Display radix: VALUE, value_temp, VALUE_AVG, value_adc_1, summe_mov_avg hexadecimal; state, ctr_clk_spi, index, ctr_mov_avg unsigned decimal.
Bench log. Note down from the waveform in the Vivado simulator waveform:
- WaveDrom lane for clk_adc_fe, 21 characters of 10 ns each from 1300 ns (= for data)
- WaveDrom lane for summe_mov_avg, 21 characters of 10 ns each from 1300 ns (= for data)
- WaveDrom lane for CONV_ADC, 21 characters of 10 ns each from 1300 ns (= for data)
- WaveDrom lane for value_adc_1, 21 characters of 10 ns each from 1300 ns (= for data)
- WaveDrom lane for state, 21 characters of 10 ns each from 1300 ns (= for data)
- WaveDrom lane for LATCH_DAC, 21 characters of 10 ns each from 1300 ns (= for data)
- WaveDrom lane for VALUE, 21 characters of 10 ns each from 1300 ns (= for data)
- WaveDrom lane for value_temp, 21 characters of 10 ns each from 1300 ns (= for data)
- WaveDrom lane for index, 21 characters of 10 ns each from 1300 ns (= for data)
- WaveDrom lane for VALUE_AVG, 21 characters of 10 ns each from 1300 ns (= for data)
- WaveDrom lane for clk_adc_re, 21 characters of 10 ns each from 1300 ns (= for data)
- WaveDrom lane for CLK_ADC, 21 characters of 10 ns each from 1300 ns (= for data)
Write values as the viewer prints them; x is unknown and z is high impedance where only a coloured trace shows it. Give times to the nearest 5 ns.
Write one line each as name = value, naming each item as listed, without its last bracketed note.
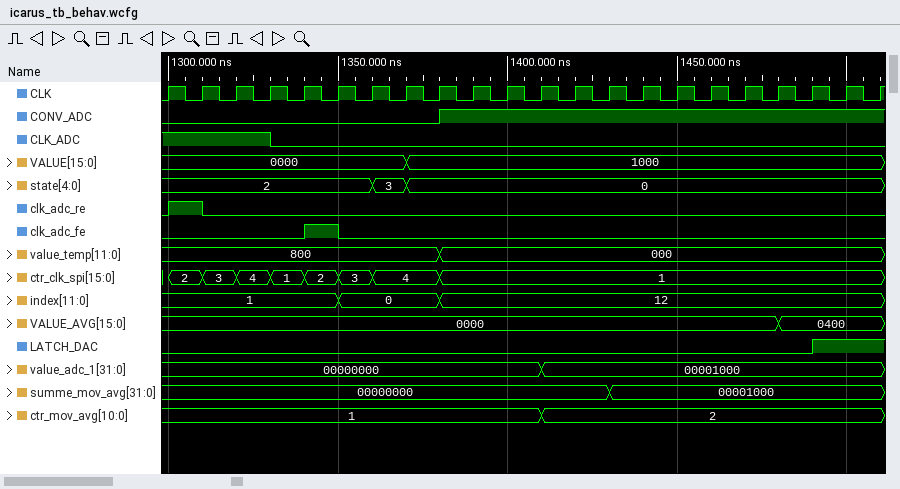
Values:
WaveDrom lane for clk_adc_fe, 21 characters of 10 ns each from 1300 ns = {name: 'clk_adc_fe', wave: '0...10...............'}
WaveDrom lane for summe_mov_avg, 21 characters of 10 ns each from 1300 ns = {name: 'summe_mov_avg', wave: '=............=.......', data: '00000000 00001000'}
WaveDrom lane for CONV_ADC, 21 characters of 10 ns each from 1300 ns = {name: 'CONV_ADC', wave: '0.......1............'}
WaveDrom lane for value_adc_1, 21 characters of 10 ns each from 1300 ns = {name: 'value_adc_1', wave: '=..........=.........', data: '00000000 00001000'}
WaveDrom lane for state, 21 characters of 10 ns each from 1300 ns = {name: 'state', wave: '=.....==.............', data: '2 3 0'}
WaveDrom lane for LATCH_DAC, 21 characters of 10 ns each from 1300 ns = {name: 'LATCH_DAC', wave: '0..................1.'}
WaveDrom lane for VALUE, 21 characters of 10 ns each from 1300 ns = {name: 'VALUE', wave: '=......=.............', data: '0000 1000'}
WaveDrom lane for value_temp, 21 characters of 10 ns each from 1300 ns = {name: 'value_temp', wave: '=.......=............', data: '800 000'}
WaveDrom lane for index, 21 characters of 10 ns each from 1300 ns = {name: 'index', wave: '=....=..=............', data: '1 0 12'}
WaveDrom lane for VALUE_AVG, 21 characters of 10 ns each from 1300 ns = {name: 'VALUE_AVG', wave: '=.................=..', data: '0000 0400'}
WaveDrom lane for clk_adc_re, 21 characters of 10 ns each from 1300 ns = {name: 'clk_adc_re', wave: '10...................'}
WaveDrom lane for CLK_ADC, 21 characters of 10 ns each from 1300 ns = {name: 'CLK_ADC', wave: '1..0.................'}
